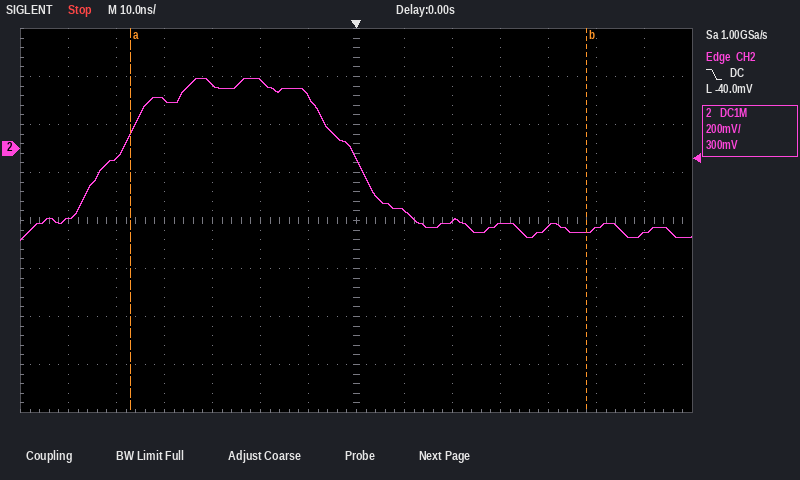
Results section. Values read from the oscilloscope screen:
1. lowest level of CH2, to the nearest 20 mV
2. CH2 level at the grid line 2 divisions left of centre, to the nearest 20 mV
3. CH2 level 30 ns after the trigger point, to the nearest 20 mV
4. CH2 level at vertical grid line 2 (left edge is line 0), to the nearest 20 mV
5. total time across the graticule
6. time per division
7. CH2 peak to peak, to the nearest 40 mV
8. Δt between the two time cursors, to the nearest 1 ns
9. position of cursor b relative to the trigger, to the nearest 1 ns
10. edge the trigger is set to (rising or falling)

-380 mV
280 mV
-320 mV
-40 mV
140 ns
10 ns
680 mV
95 ns
+48 ns
falling
